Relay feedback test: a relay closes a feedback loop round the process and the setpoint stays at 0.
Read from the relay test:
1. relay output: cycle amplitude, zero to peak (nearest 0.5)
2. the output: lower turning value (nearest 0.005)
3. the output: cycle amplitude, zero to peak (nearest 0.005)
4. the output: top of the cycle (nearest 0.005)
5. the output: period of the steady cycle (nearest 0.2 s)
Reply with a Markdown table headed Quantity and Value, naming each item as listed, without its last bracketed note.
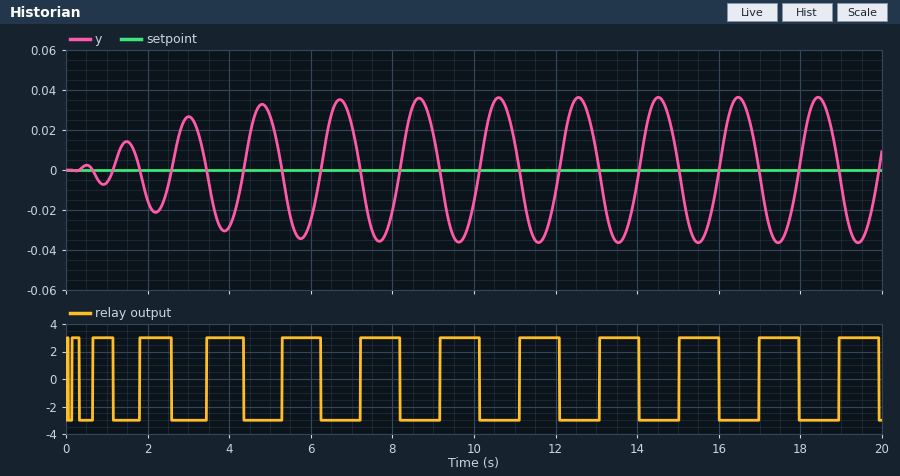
| Quantity | Value |
|---|---|
| relay output: cycle amplitude, zero to peak | 3.0 |
| the output: lower turning value | -0.035 |
| the output: cycle amplitude, zero to peak | 0.035 |
| the output: top of the cycle | 0.035 |
| the output: period of the steady cycle | 2.0 s |
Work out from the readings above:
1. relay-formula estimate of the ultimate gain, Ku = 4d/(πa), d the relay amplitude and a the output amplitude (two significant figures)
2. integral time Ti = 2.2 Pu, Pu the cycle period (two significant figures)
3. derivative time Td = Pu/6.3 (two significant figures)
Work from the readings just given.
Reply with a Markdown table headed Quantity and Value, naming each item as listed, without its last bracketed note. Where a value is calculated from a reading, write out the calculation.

| Quantity | Value |
|---|---|
| relay-formula estimate of the ultimate gain, Ku = 4d/(πa), d the relay amplitude and a the output amplitude | 4 × 3 / (π × 0.035) = 110 |
| integral time Ti = 2.2 Pu, Pu the cycle period | 2.2 × 2 = 4.4 s |
| derivative time Td = Pu/6.3 | 2 / 6.3 = 0.32 s |
